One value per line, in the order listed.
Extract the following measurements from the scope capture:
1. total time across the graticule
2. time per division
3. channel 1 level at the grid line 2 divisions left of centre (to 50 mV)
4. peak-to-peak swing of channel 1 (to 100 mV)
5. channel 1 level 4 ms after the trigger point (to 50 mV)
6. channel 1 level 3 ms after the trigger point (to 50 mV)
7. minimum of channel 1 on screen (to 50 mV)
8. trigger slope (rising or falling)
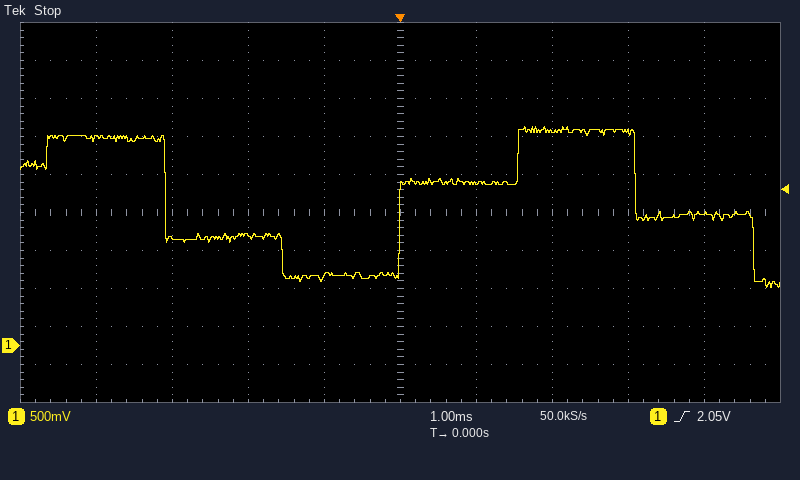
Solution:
10 ms
1 ms
1.45 V
2.10 V
1.75 V
2.80 V
750 mV
rising
